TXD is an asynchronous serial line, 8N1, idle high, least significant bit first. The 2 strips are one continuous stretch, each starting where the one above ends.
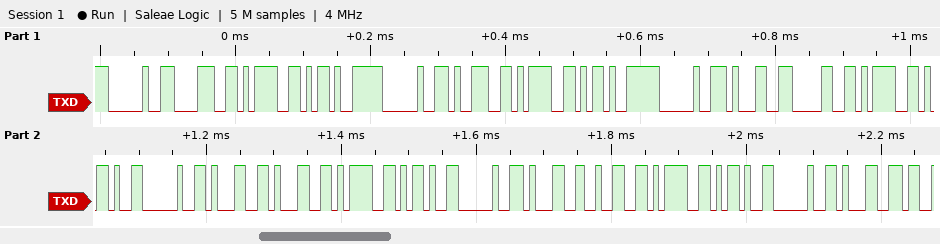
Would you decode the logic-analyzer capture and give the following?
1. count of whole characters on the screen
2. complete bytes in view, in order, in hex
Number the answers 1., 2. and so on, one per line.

1. 25
2. 0x20 0x38 0x3D 0x2D 0x20 0x39 0x3D 0x2D 0x20 0x31 0x30 0x3D 0x2D 0x20 0x31 0x31 0x3D 0x2D 0x20 0x31 0x32 0x3D 0x2D 0x20 0x31
